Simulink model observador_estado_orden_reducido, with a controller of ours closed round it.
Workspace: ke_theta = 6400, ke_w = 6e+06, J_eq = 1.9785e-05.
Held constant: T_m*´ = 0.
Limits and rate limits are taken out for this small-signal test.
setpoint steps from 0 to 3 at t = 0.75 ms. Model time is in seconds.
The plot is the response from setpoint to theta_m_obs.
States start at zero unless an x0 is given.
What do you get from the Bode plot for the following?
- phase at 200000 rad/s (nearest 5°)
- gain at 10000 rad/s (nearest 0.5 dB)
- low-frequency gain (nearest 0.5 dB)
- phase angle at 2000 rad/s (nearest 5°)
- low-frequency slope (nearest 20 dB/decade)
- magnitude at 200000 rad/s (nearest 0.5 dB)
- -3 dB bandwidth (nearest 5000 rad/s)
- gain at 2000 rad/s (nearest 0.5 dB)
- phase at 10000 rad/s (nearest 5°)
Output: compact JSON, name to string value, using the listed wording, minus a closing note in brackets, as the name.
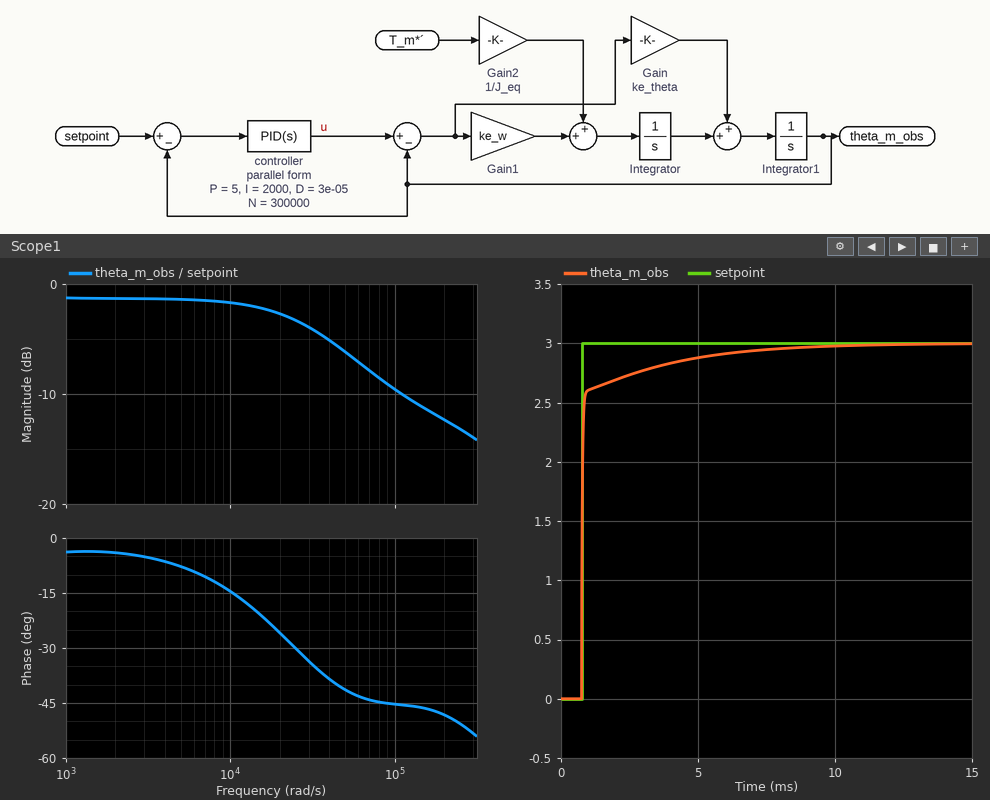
{"phase at 200000 rad/s": "-50°", "gain at 10000 rad/s": "-1.5 dB", "low-frequency gain": "-1.5 dB", "phase angle at 2000 rad/s": "-5°", "low-frequency slope": "0 dB/decade", "magnitude at 200000 rad/s": "-12.5 dB", "-3 dB bandwidth": "35000 rad/s", "gain at 2000 rad/s": "-1.5 dB", "phase at 10000 rad/s": "-15°"}
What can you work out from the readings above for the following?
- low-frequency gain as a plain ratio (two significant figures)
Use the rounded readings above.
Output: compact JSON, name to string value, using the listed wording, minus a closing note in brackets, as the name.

{"low-frequency gain as a plain ratio": "0.84"}
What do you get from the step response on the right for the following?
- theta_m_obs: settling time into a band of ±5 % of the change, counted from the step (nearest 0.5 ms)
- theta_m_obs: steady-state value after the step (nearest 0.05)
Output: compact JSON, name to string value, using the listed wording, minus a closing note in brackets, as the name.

{"theta_m_obs: settling time into a band of ±5 % of the change, counted from the step": "3.5 ms", "theta_m_obs: steady-state value after the step": "3.00"}
